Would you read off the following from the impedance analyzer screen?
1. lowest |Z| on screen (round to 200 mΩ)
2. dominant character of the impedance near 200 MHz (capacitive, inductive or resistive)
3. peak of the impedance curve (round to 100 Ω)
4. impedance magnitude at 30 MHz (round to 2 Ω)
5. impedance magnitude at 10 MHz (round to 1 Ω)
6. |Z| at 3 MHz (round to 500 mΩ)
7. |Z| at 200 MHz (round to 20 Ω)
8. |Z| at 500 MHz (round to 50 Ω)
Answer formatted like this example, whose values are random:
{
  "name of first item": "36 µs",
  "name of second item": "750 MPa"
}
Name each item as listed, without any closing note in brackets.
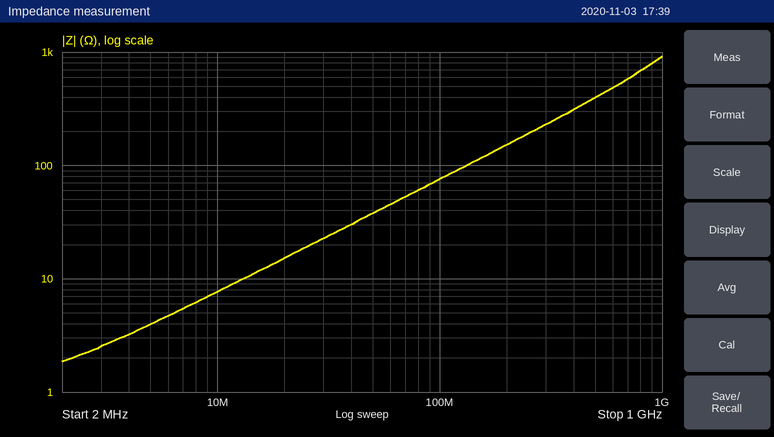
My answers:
{
  "lowest |Z| on screen": "1.8 Ω",
  "dominant character of the impedance near 200 MHz": "inductive",
  "peak of the impedance curve": "900 Ω",
  "impedance magnitude at 30 MHz": "22 Ω",
  "impedance magnitude at 10 MHz": "8 Ω",
  "|Z| at 3 MHz": "2.5 Ω",
  "|Z| at 200 MHz": "160 Ω",
  "|Z| at 500 MHz": "400 Ω"
}
